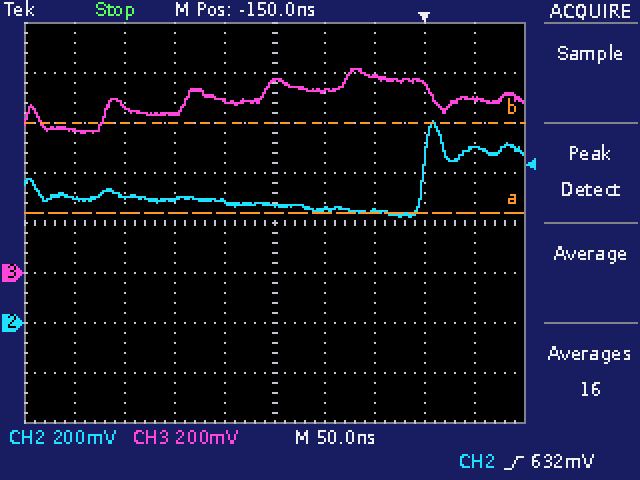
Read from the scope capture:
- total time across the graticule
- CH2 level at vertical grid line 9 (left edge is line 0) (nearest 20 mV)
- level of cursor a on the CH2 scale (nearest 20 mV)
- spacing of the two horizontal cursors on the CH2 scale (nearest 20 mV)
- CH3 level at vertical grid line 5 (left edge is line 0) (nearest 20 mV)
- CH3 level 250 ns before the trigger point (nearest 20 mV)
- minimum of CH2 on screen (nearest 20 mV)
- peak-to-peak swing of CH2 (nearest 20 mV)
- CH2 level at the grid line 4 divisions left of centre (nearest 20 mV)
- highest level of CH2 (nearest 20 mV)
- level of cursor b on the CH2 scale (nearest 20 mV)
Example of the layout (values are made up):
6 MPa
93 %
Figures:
500 ns
700 mV
440 mV
360 mV
760 mV
640 mV
420 mV
380 mV
500 mV
800 mV
800 mV
